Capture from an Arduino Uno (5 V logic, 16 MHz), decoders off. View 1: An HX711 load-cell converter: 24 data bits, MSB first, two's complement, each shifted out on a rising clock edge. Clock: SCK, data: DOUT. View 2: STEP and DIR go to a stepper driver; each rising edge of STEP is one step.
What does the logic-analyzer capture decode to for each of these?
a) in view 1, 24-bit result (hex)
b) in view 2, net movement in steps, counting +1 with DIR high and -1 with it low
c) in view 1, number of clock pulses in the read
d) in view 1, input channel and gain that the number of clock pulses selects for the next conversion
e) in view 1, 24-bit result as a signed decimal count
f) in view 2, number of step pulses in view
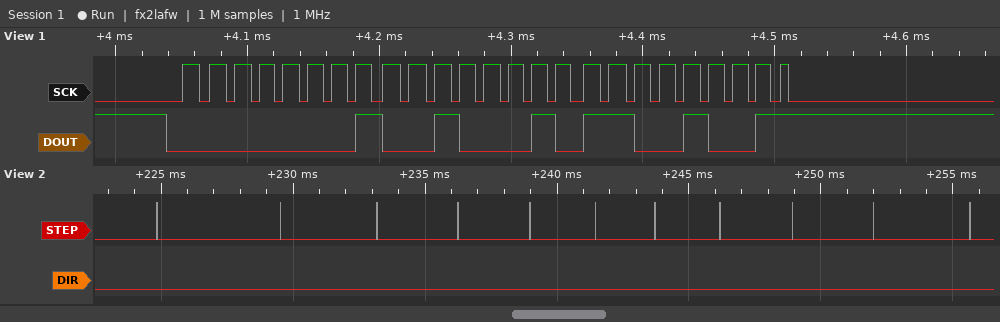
0x0122C9
-11
25
channel A, gain 128
74441
11
